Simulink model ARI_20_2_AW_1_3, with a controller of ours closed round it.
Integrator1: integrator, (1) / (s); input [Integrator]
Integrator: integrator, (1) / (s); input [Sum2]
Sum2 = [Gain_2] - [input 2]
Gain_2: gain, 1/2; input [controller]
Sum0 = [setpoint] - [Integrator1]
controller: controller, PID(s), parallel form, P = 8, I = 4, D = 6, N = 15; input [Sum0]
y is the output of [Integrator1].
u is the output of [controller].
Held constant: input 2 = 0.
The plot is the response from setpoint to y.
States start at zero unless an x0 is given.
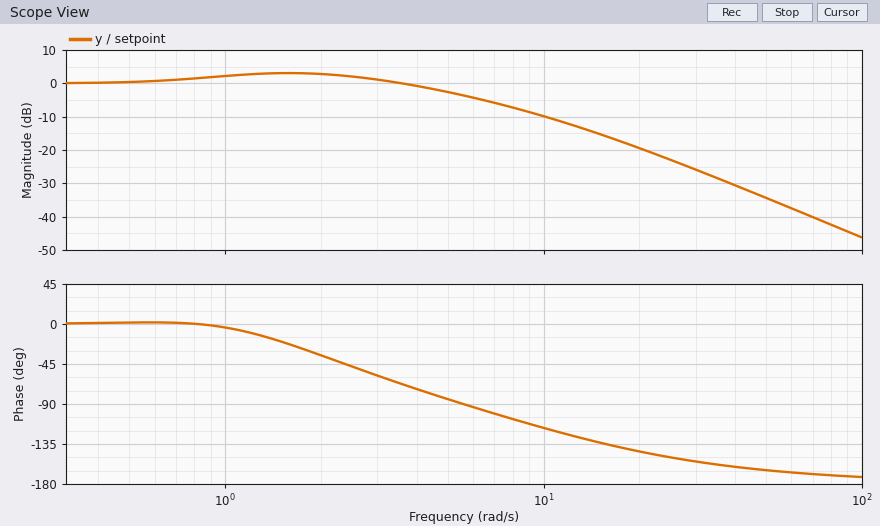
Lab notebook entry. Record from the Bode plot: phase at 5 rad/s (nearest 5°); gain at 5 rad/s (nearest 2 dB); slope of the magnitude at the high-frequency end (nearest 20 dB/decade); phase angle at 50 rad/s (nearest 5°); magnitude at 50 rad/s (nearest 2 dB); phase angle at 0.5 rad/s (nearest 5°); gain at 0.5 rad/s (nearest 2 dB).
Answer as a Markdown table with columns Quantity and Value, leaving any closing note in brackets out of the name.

| Quantity | Value |
|---|---|
| phase at 5 rad/s | -85° |
| gain at 5 rad/s | -2 dB |
| slope of the magnitude at the high-frequency end | -40 dB/decade |
| phase angle at 50 rad/s | -165° |
| magnitude at 50 rad/s | -34 dB |
| phase angle at 0.5 rad/s | 0° |
| gain at 0.5 rad/s | 0 dB |
